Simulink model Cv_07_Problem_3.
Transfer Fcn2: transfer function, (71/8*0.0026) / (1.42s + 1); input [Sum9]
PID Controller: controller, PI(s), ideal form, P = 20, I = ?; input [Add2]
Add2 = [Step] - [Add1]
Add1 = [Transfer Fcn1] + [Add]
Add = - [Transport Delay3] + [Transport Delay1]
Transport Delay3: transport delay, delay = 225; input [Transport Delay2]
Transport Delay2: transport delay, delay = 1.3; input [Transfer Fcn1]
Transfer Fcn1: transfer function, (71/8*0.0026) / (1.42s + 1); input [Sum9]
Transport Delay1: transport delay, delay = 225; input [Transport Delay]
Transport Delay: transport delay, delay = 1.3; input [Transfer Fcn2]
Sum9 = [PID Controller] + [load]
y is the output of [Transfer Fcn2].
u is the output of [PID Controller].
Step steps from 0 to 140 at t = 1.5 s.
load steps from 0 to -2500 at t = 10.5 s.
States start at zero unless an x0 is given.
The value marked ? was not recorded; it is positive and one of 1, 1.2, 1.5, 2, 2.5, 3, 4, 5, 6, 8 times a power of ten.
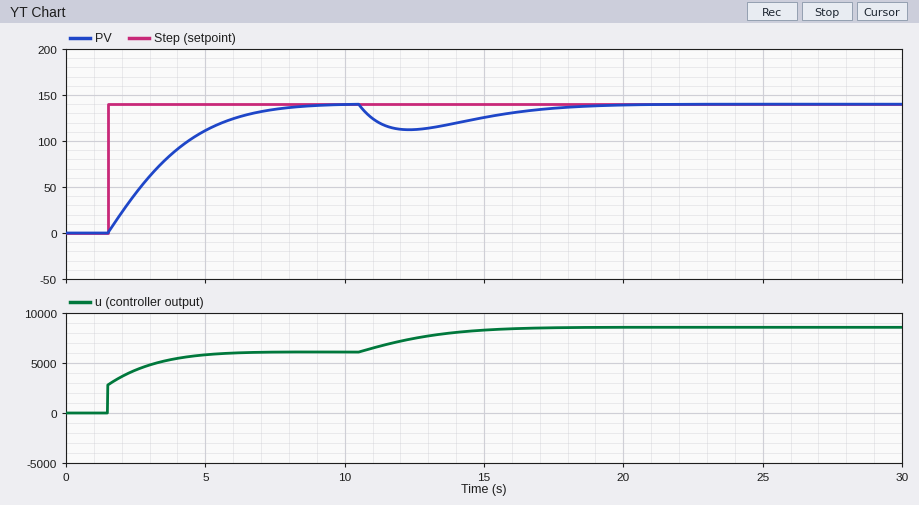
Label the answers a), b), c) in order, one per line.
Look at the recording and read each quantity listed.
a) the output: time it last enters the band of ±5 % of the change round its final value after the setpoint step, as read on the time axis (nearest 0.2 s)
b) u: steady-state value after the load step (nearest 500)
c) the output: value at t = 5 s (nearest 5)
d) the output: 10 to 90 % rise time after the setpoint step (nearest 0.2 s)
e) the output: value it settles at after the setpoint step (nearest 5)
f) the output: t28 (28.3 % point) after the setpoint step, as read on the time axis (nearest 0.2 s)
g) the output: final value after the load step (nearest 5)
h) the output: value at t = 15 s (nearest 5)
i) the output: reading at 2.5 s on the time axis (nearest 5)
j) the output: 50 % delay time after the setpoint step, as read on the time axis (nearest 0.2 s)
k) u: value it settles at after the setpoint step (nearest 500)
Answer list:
a) 7.2 s
b) 8500
c) 110
d) 4.4 s
e) 140
f) 2.4 s
g) 140
h) 125
i) 45
j) 3.2 s
k) 6000
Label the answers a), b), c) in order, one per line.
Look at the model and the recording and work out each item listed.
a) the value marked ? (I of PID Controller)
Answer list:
a) 1
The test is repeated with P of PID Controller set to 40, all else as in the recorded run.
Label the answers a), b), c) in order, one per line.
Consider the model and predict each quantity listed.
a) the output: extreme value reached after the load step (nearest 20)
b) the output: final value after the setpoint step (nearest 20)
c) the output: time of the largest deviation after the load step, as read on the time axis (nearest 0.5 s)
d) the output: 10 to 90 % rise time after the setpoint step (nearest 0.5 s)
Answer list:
a) 120
b) 140
c) 12.0 s
d) 2.5 s
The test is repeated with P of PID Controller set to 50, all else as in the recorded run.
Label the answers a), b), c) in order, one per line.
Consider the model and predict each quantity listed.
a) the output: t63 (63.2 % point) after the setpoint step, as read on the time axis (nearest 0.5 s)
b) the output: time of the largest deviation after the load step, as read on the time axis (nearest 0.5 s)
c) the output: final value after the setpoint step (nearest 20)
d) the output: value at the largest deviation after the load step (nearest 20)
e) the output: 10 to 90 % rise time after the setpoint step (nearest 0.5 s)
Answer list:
a) 2.5 s
b) 11.5 s
c) 140
d) 120
e) 2.0 s
